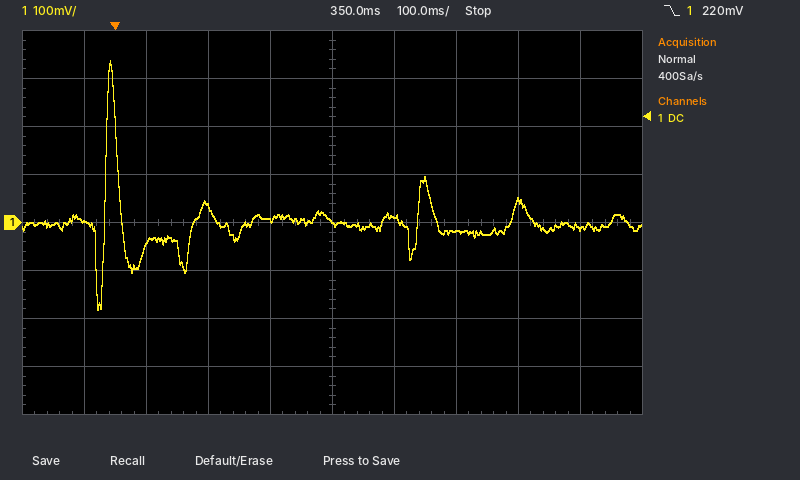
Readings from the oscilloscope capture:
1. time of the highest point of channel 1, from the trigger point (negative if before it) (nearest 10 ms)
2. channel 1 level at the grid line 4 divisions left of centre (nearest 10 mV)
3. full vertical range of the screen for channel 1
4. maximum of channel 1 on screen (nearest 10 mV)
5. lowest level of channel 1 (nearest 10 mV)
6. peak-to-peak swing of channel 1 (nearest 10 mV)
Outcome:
-10 ms
0 mV
800 mV
340 mV
-180 mV
520 mV
